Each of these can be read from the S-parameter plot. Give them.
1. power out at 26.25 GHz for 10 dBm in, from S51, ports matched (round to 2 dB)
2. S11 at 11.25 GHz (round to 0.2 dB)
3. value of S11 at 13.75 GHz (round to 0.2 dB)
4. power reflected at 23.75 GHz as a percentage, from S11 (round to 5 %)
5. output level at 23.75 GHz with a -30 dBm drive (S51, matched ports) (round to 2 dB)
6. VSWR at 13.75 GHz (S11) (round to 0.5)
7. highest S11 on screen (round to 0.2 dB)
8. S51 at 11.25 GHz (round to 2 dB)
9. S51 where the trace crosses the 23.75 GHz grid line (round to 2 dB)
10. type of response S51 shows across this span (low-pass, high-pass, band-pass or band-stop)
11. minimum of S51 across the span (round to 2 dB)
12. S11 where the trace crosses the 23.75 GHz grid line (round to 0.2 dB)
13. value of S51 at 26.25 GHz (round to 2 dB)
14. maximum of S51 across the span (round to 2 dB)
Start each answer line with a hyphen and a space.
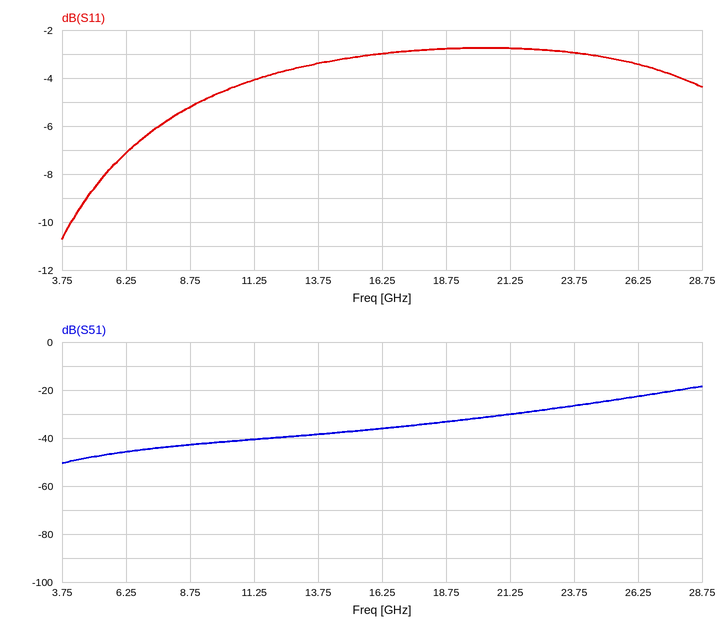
- -12 dBm
- -4.0 dB
- -3.4 dB
- 50 %
- -56 dBm
- 5.0
- -2.8 dB
- -40 dB
- -26 dB
- high-pass
- -50 dB
- -3.0 dB
- -22 dB
- -18 dB
